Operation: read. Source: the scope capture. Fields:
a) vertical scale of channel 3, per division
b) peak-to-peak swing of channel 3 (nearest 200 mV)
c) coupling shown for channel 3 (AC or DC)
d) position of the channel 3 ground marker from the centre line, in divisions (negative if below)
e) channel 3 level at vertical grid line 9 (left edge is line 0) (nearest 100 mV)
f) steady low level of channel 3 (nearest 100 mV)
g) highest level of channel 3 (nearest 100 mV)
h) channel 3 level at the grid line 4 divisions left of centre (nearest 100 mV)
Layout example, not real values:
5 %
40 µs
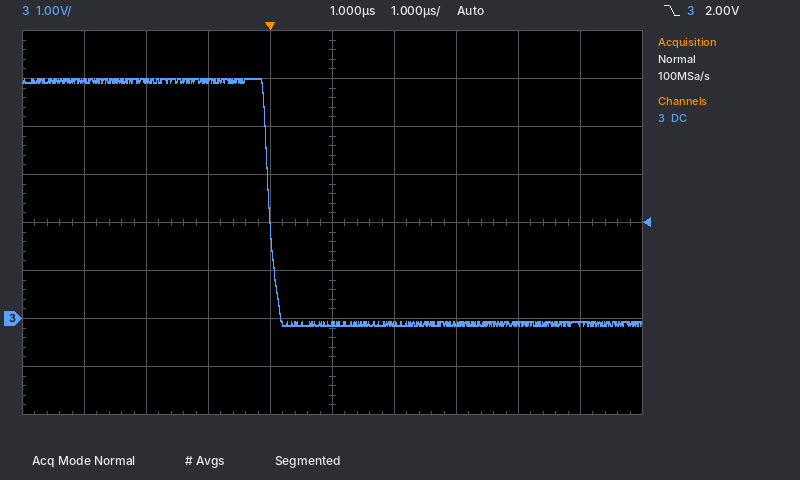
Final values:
1 V
5.2 V
DC
-2.0 div
-100 mV
-100 mV
5.0 V
5.0 V
